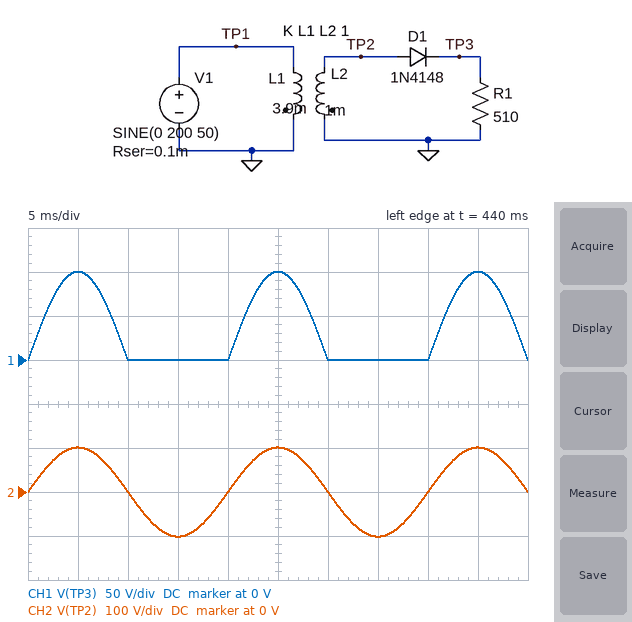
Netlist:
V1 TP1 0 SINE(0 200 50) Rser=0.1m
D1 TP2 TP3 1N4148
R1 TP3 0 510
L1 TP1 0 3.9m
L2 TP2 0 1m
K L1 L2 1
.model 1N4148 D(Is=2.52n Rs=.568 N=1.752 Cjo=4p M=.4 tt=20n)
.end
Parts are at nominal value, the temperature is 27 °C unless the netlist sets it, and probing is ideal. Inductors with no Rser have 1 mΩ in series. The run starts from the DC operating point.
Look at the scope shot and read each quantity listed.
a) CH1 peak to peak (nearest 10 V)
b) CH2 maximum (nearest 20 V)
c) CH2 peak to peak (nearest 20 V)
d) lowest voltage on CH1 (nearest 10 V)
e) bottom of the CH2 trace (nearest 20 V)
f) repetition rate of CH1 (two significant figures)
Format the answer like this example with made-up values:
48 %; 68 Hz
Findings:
100 V; 100 V; 200 V; 0 V; -100 V; 50 Hz
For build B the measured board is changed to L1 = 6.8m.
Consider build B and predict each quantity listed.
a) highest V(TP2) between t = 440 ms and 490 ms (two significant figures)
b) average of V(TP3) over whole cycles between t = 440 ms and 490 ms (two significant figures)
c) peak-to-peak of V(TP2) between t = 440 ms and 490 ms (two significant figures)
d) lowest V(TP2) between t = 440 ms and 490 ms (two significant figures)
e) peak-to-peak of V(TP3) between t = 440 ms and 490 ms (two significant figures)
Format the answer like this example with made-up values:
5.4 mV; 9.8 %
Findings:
77 V; 24 V; 150 V; -77 V; 76 V
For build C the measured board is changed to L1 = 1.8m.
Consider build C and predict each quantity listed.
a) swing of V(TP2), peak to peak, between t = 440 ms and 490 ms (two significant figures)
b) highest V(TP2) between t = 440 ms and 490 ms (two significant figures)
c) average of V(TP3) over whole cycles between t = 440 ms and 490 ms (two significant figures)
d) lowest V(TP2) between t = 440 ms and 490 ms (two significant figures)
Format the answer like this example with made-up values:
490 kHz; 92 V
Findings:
300 V; 150 V; 47 V; -150 V
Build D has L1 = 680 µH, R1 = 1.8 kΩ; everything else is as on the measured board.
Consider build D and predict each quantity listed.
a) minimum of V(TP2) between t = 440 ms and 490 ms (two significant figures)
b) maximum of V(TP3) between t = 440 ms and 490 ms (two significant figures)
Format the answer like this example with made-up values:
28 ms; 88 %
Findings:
-240 V; 240 V
